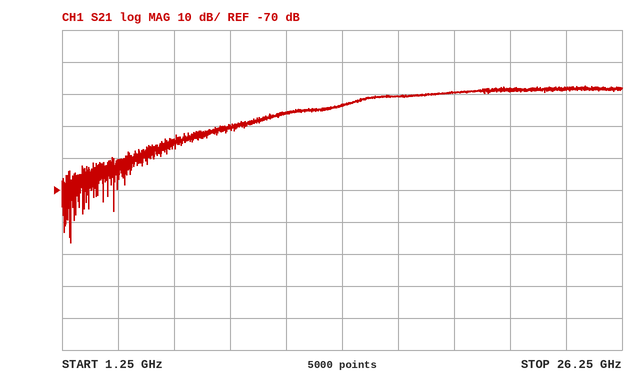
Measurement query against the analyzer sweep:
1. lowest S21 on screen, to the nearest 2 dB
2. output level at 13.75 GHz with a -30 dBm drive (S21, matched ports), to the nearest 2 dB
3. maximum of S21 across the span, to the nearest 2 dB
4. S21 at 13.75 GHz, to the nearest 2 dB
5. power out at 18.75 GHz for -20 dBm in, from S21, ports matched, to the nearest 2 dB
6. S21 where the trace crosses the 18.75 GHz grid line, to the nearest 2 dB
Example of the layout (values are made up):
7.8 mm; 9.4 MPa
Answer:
-86 dB; -74 dBm; -38 dB; -44 dB; -60 dBm; -40 dB
